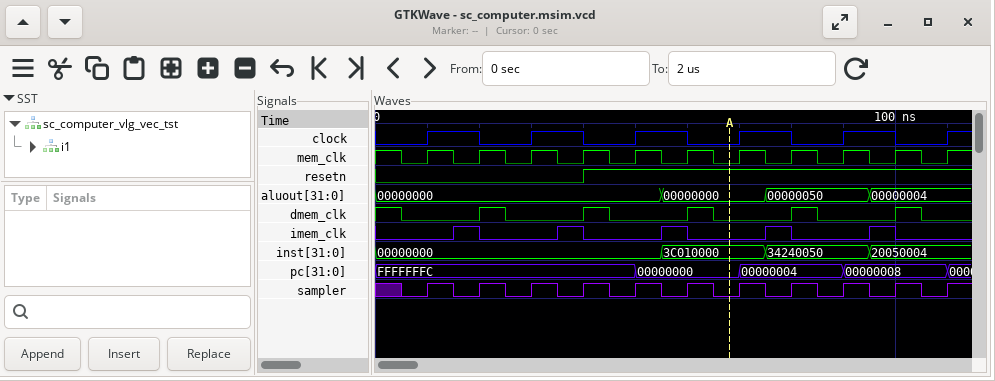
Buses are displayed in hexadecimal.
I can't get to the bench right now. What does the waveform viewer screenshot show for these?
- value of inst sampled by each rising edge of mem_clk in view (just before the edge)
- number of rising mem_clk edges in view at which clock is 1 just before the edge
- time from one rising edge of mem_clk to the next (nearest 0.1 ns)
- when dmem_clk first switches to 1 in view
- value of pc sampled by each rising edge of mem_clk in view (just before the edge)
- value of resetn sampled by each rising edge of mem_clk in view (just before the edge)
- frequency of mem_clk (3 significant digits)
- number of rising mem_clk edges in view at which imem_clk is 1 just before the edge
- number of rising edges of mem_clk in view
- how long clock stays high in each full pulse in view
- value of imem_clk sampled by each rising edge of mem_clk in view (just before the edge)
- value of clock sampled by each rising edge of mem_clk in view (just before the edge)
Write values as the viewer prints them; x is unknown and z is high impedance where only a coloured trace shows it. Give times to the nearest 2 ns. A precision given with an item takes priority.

00000000, 00000000, 00000000, 00000000, 00000000, 3C010000, 3C010000, 34240050, 34240050, 20050004, 20050004
5
10 ns
20 ns
FFFFFFFC, FFFFFFFC, FFFFFFFC, FFFFFFFC, FFFFFFFC, 00000000, 00000000, 00000004, 00000004, 00000008, 00000008
0 0 0 0 1 1 1 1 1 1 1
100 MHz
5
11
10 ns, 10 ns, 10 ns, 10 ns, 10 ns
0 1 0 1 0 1 0 1 0 1 0
0 1 0 1 0 1 0 1 0 1 0
